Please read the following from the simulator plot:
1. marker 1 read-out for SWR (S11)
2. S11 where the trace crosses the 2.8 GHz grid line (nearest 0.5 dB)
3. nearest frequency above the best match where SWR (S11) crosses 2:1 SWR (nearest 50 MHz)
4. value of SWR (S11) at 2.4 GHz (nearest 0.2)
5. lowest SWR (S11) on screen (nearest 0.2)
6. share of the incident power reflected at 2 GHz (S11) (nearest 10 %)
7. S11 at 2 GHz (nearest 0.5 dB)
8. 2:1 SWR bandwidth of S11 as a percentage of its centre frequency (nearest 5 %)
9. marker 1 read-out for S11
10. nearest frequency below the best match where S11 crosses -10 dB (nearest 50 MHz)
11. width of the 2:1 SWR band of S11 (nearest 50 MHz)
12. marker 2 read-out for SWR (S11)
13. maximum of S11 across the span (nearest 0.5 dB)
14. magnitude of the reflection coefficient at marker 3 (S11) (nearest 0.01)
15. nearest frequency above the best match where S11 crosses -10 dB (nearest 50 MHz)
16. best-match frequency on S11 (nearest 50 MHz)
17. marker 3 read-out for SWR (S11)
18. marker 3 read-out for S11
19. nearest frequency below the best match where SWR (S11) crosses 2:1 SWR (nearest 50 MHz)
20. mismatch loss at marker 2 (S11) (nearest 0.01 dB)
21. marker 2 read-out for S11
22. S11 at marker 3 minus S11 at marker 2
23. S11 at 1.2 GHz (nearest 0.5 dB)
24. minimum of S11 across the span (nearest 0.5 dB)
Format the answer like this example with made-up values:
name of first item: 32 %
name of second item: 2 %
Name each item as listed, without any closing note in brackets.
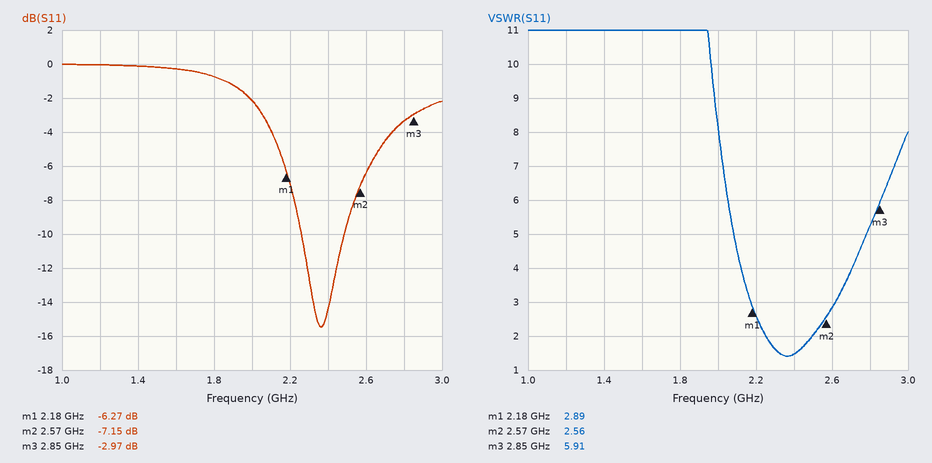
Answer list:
marker 1 read-out for SWR: 2.89
S11 where the trace crosses the 2.8 GHz grid line: -3.5 dB
nearest frequency above the best match where SWR (S11) crosses 2:1 SWR: 2.50 GHz
value of SWR (S11) at 2.4 GHz: 1.4
lowest SWR (S11) on screen: 1.4
share of the incident power reflected at 2 GHz (S11): 60 %
S11 at 2 GHz: -2.0 dB
2:1 SWR bandwidth of S11 as a percentage of its centre frequency: 10 %
marker 1 read-out for S11: -6.27 dB
nearest frequency below the best match where S11 crosses -10 dB: 2.25 GHz
width of the 2:1 SWR band of S11: 250 MHz
marker 2 read-out for SWR: 2.56
maximum of S11 across the span: 0.0 dB
magnitude of the reflection coefficient at marker 3 (S11): 0.71
nearest frequency above the best match where S11 crosses -10 dB: 2.50 GHz
best-match frequency on S11: 2.35 GHz
marker 3 read-out for SWR: 5.91
marker 3 read-out for S11: -2.97 dB
nearest frequency below the best match where SWR (S11) crosses 2:1 SWR: 2.25 GHz
mismatch loss at marker 2 (S11): 0.93 dB
marker 2 read-out for S11: -7.15 dB
S11 at marker 3 minus S11 at marker 2: 4.18 dB
S11 at 1.2 GHz: 0.0 dB
minimum of S11 across the span: -15.5 dB
